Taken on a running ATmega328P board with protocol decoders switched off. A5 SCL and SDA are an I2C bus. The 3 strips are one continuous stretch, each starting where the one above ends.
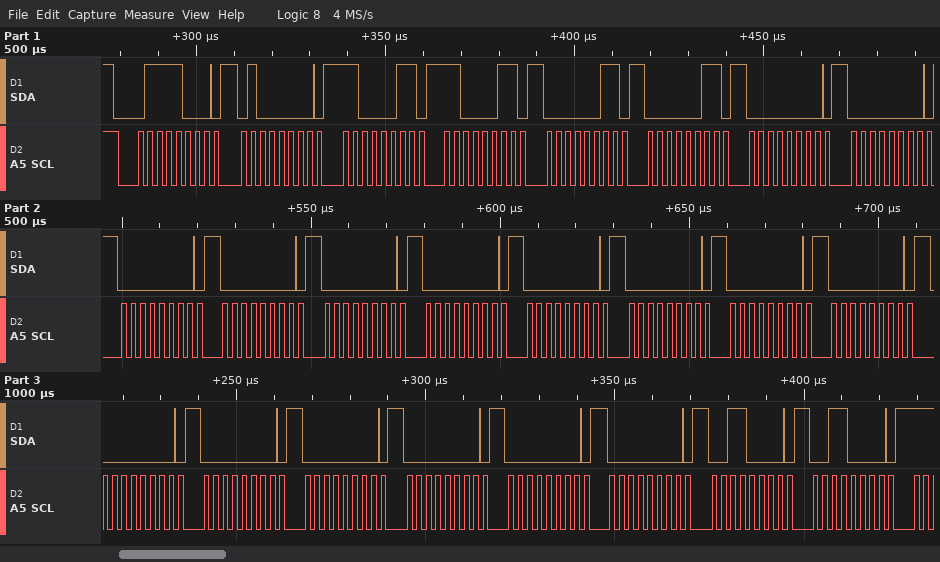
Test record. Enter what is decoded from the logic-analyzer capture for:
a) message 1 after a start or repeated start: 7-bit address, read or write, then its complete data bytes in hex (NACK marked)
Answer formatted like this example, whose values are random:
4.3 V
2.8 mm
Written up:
0x3C write: 40 C3 C3 03 03 00 00 00 00 00 00 00 00 00 00 00 00 00 00 00 00 30 30
